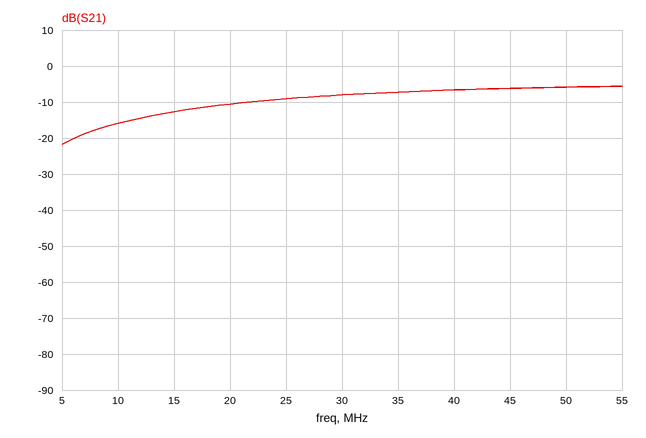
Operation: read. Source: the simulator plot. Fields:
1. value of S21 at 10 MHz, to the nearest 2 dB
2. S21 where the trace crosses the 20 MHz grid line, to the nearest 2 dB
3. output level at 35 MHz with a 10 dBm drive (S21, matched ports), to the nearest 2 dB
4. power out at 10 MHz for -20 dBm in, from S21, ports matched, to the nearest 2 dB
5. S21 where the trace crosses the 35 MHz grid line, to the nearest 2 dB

-16 dB
-10 dB
2 dBm
-36 dBm
-8 dB
